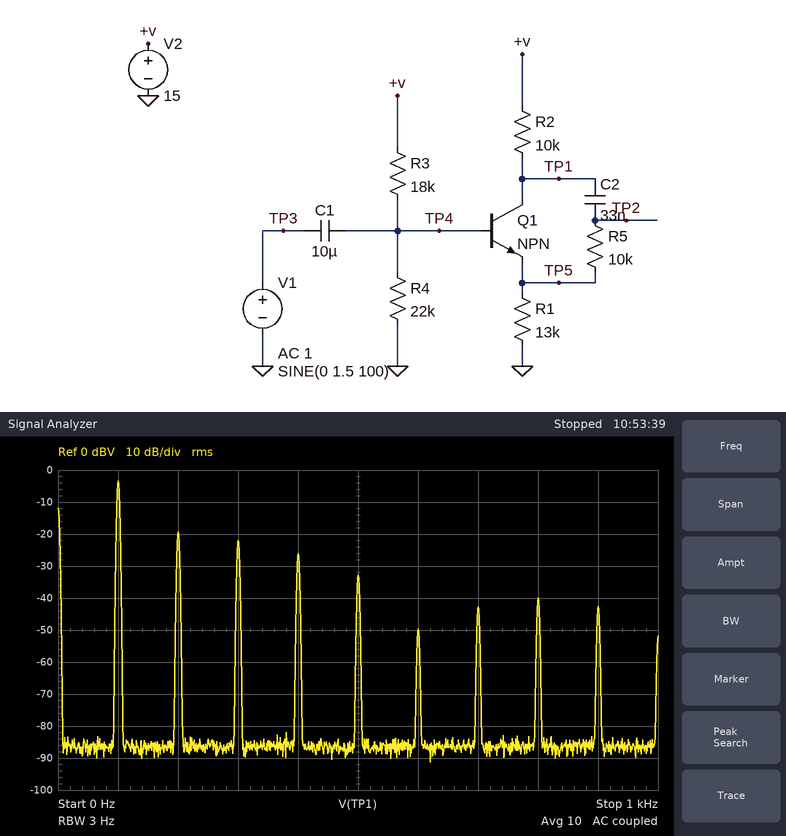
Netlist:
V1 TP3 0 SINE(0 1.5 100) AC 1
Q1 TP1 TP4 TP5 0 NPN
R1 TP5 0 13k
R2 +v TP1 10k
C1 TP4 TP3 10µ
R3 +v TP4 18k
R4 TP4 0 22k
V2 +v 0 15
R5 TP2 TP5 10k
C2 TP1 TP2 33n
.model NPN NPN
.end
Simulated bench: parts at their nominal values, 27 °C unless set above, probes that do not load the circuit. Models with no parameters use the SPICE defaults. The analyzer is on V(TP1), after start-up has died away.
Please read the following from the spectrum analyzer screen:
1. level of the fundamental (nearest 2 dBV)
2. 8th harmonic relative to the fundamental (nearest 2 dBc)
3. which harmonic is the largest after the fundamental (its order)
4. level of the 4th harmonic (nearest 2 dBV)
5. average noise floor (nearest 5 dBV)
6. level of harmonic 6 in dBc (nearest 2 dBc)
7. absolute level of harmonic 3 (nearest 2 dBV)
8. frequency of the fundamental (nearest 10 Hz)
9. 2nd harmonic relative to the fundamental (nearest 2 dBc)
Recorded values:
-4 dBV
-36 dBc
2
-26 dBV
-85 dBV
-46 dBc
-22 dBV
100 Hz
-16 dBc
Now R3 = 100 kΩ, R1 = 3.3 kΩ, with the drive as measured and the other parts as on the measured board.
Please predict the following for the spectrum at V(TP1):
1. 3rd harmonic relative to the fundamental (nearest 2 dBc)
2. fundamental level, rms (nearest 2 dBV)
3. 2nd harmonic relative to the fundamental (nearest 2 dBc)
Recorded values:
-54 dBc
10 dBV
-46 dBc
